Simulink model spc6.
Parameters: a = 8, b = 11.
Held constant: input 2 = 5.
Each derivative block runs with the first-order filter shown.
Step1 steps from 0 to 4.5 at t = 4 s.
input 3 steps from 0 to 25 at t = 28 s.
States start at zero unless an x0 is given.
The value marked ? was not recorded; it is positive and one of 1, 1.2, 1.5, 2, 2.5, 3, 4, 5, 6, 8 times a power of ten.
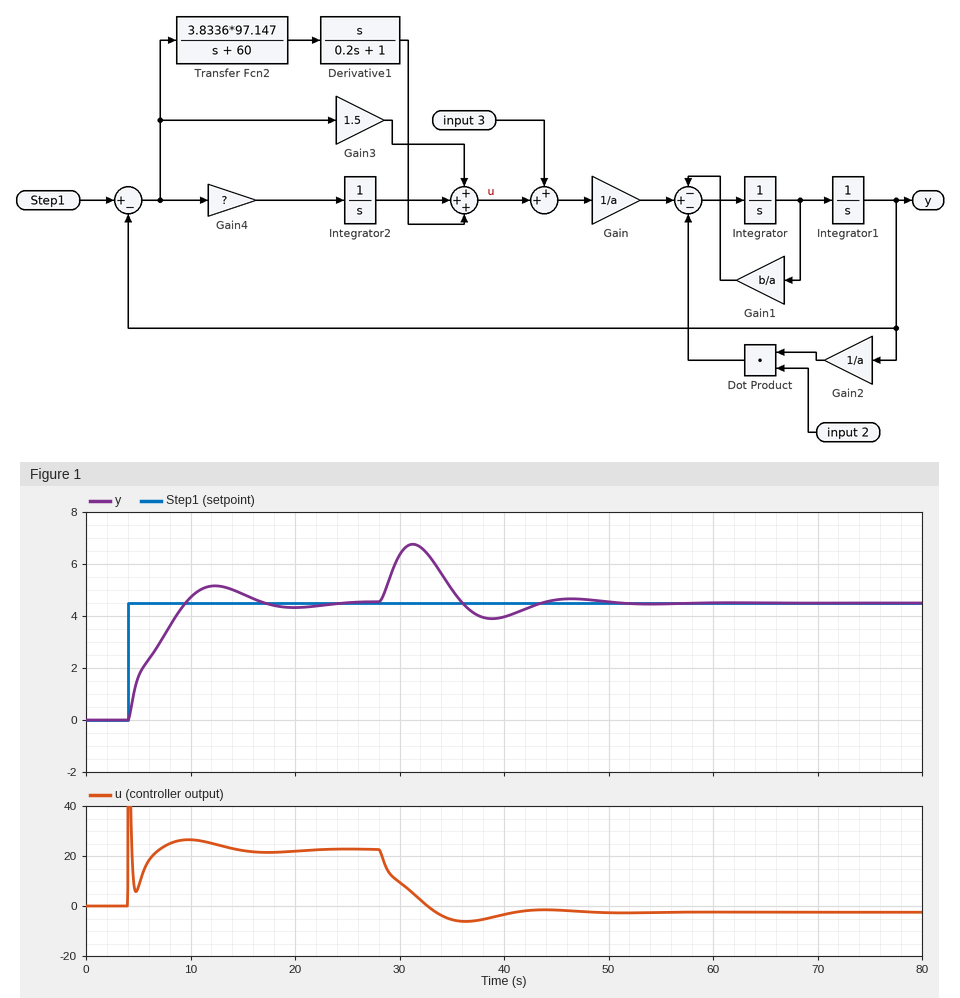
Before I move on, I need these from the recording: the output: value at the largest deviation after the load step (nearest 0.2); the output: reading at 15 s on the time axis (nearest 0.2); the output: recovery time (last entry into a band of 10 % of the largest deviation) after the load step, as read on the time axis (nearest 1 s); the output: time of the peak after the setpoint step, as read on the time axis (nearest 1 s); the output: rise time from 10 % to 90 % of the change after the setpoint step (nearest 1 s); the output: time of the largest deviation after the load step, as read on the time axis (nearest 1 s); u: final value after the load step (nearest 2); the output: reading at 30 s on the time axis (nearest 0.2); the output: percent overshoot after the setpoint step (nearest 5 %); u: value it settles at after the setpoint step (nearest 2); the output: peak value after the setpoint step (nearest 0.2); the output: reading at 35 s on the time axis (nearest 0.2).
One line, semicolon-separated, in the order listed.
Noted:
6.8; 4.8; 42 s; 12 s; 4 s; 31 s; -2; 6.4; 15 %; 22; 5.2; 5.0
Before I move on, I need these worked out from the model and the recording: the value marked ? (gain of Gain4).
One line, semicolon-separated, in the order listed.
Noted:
3
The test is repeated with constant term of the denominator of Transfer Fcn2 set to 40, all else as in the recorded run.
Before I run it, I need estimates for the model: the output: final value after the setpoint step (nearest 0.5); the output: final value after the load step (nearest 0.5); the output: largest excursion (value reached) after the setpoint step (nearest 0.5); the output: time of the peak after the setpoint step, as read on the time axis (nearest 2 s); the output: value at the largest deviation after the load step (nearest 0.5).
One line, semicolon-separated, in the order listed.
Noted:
4.5; 4.5; 5.0; 14 s; 6.5
